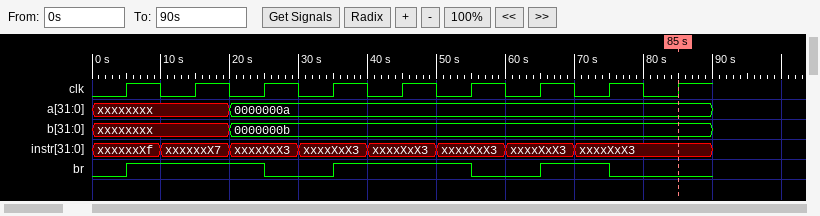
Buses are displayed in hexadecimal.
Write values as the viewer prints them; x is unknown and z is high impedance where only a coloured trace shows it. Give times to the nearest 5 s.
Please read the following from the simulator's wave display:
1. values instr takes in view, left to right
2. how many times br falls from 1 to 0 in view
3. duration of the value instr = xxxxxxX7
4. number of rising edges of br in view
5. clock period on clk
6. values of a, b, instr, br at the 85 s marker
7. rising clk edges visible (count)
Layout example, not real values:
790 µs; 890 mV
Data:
xxxxxxXf, xxxxxxX7, xxxxXxX3, xxxxXxX3, xxxxXxX3, xxxxXxX3, xxxxXxX3, xxxxXxX3; 3; 10 s; 3; 10 s; a=0000000a, b=0000000b, instr=xxxxXxX3, br=0; 9
